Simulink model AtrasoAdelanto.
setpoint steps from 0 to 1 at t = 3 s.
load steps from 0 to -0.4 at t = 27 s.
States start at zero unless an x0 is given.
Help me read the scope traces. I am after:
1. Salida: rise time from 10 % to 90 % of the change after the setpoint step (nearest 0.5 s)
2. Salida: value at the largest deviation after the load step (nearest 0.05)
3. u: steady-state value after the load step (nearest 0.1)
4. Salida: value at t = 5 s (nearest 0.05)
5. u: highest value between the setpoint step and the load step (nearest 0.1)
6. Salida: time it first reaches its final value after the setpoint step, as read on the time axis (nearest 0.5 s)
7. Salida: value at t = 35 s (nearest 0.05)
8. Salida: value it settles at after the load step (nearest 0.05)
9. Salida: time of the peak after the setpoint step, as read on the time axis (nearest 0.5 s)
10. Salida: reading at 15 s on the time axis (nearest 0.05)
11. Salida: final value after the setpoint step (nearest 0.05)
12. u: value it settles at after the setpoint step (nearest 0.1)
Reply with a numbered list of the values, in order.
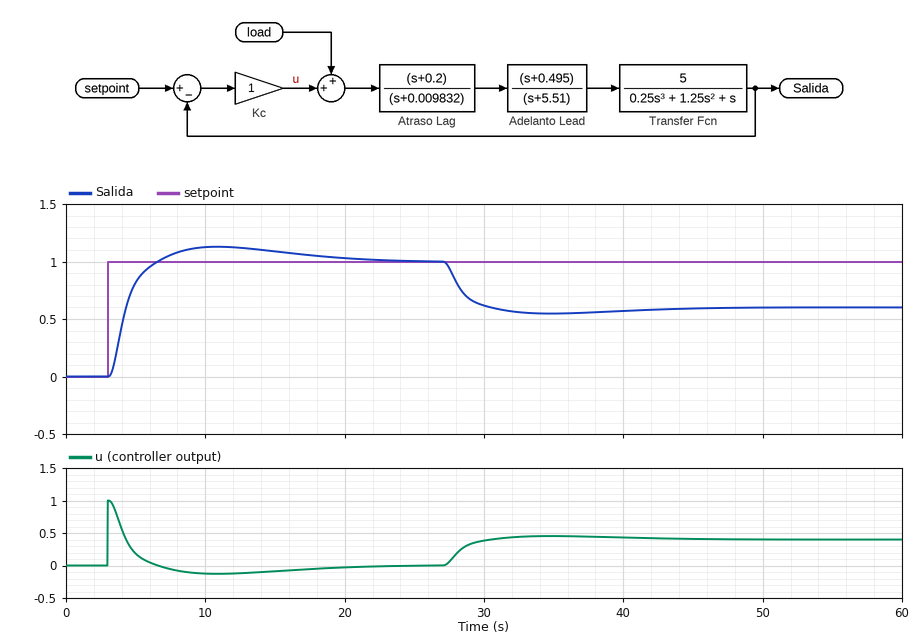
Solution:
1. 2.0 s
2. 0.55
3. 0.4
4. 0.80
5. 1.0
6. 6.5 s
7. 0.55
8. 0.60
9. 11.0 s
10. 1.10
11. 1.00
12. 0.0
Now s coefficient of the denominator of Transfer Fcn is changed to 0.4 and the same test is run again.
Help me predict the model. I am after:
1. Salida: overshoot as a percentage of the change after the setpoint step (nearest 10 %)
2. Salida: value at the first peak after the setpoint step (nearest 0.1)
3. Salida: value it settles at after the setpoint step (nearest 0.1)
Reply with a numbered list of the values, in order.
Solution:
1. 30 %
2. 1.3
3. 1.0
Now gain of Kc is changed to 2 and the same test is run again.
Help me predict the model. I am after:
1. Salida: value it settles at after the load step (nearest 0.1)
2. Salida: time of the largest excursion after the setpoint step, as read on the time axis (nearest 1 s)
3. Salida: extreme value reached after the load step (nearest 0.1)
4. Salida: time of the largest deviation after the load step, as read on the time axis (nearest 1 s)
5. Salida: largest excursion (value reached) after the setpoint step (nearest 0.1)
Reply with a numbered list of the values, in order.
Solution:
1. 0.8
2. 9 s
3. 0.8
4. 33 s
5. 1.1
